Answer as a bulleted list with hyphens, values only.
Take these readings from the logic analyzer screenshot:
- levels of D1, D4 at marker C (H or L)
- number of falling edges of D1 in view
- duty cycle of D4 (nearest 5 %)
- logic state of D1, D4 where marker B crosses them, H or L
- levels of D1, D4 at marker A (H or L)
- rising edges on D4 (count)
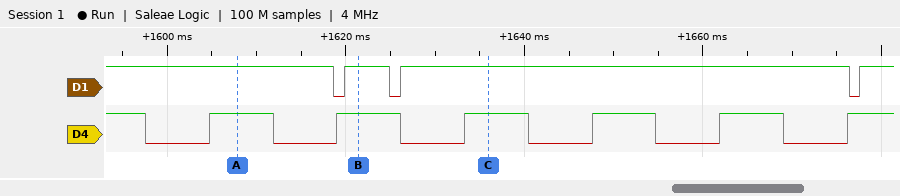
- D1=H, D4=H
- 3
- 50 %
- D1=H, D4=H
- D1=H, D4=H
- 6
